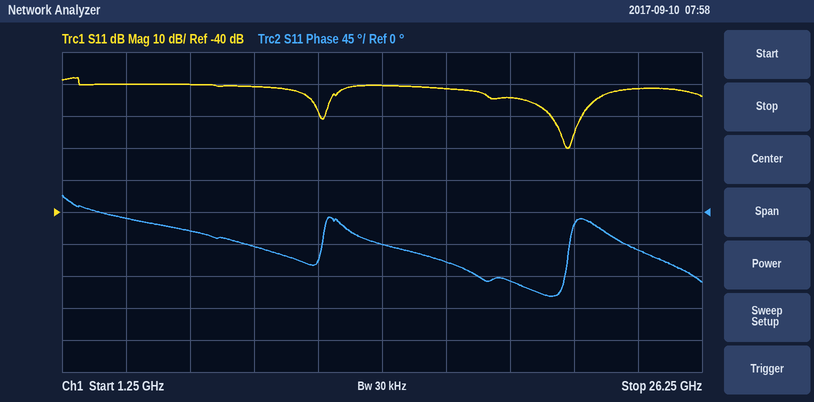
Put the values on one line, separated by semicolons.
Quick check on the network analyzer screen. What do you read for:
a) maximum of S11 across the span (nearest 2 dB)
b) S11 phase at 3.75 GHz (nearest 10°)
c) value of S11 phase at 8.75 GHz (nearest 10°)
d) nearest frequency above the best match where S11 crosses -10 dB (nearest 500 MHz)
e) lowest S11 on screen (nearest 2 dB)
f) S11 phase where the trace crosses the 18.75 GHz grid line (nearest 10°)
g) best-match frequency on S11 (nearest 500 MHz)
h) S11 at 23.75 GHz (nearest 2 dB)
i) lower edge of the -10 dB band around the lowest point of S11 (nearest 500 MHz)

2 dB; -10°; -50°; 21.5 GHz; -20 dB; -100°; 21.0 GHz; -2 dB; 20.5 GHz
